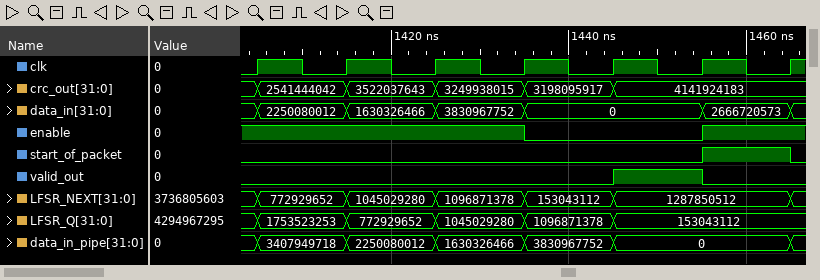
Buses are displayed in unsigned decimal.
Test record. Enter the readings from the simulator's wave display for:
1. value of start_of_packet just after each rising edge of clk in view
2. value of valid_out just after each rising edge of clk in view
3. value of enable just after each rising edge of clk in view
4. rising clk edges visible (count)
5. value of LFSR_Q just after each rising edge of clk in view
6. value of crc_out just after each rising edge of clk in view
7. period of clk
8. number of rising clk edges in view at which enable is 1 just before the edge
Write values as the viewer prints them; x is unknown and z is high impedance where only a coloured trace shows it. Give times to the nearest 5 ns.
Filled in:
0 0 0 0 0 1 0
0 0 0 0 1 0 0
1 1 1 0 0 1 1
7
1753523253, 772929652, 1045029280, 1096871378, 153043112, 153043112, 153043112
2541444042, 3522037643, 3249938015, 3198095917, 4141924183, 4141924183, 4141924183
10 ns
5
